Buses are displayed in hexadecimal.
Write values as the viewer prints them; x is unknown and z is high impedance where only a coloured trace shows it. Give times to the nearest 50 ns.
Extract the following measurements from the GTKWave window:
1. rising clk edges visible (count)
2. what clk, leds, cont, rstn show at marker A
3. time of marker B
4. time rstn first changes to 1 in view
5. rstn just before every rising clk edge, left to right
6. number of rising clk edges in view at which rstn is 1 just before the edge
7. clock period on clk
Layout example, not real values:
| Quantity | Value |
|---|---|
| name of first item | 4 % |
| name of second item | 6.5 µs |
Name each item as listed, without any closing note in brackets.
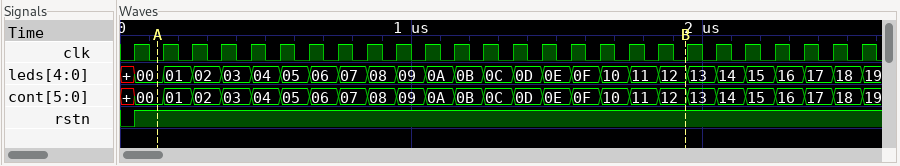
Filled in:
| Quantity | Value |
|---|---|
| rising clk edges visible | 26 |
| what clk, leds, cont, rstn show at marker A | clk=0, leds=00, cont=00, rstn=1 |
| time of marker B | 1950 ns |
| time rstn first changes to 1 in view | 50 ns |
| rstn just before every rising clk edge, left to right | 0 1 1 1 1 1 1 1 1 1 1 1 1 1 1 1 1 1 1 1 1 1 1 1 1 1 |
| number of rising clk edges in view at which rstn is 1 just before the edge | 25 |
| clock period on clk | 100 ns |
